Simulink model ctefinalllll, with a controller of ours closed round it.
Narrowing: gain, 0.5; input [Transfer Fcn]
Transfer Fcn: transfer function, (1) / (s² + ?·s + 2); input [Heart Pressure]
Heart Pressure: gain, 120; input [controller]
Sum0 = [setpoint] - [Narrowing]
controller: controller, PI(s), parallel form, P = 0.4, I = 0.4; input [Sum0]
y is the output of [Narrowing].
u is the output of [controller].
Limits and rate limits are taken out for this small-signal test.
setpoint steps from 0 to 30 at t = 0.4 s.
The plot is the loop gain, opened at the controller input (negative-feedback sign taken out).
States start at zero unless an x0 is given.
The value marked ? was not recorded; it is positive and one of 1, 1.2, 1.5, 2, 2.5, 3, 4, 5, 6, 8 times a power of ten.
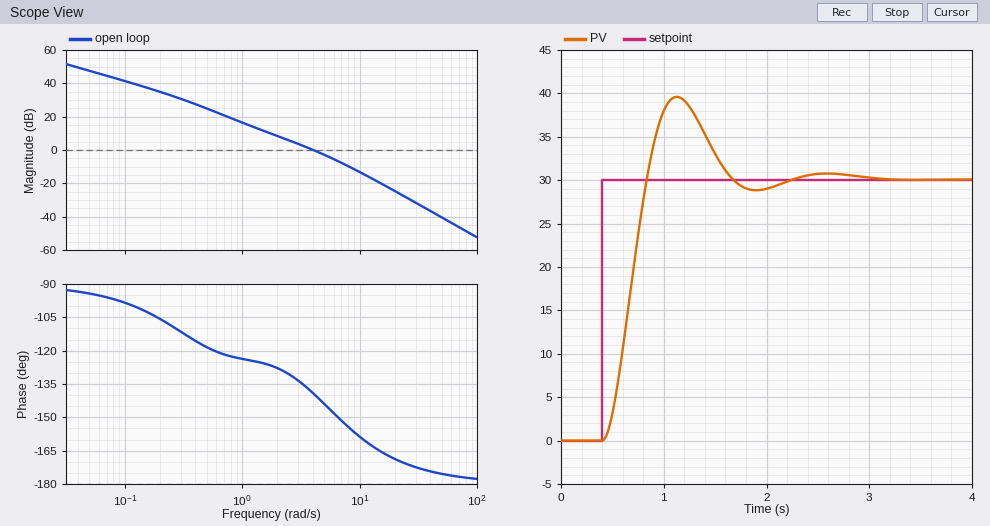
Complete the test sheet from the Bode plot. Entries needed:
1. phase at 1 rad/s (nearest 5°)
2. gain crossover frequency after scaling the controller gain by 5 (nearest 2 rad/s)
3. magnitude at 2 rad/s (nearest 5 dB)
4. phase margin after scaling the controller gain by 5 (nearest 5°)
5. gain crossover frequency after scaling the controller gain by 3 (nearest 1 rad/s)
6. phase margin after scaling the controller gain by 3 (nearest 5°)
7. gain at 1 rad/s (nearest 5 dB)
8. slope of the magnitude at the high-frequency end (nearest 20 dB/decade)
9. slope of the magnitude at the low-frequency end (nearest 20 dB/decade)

-125°
10 rad/s
10 dB
20°
8 rad/s
25°
15 dB
-40 dB/decade
-20 dB/decade
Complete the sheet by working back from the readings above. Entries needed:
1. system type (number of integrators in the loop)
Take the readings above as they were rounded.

1
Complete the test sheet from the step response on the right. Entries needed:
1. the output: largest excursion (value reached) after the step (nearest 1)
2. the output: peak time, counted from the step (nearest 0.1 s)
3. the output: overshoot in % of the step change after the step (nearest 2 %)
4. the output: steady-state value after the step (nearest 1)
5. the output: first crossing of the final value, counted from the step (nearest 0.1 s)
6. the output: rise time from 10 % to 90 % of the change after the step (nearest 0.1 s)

40
0.7 s
32 %
30
0.4 s
0.3 s
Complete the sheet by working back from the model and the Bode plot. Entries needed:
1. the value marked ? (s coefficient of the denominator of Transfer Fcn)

5
